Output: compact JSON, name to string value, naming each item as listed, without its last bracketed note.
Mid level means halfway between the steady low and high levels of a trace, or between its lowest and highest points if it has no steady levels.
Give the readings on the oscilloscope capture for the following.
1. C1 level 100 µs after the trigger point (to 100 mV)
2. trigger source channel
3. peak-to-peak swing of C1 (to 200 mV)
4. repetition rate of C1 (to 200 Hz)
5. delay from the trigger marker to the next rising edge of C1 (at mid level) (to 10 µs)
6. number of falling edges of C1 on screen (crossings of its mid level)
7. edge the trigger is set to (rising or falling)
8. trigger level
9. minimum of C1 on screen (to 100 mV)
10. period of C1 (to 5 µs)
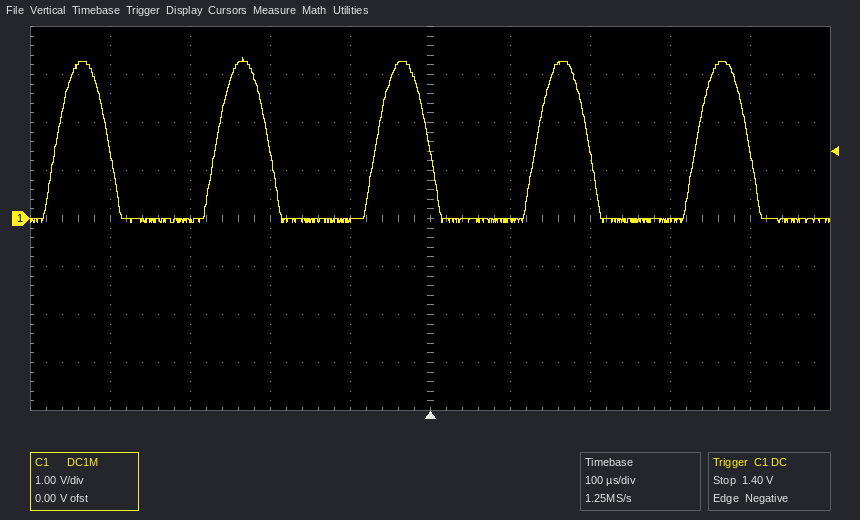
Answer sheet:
{"C1 level 100 µs after the trigger point": "0.0 V", "trigger source channel": "C1", "peak-to-peak swing of C1": "3.4 V", "repetition rate of C1": "5.0 kHz", "delay from the trigger marker to the next rising edge of C1 (at mid level)": "130 µs", "number of falling edges of C1 on screen": "5", "edge the trigger is set to": "falling", "trigger level": "1.40 V", "minimum of C1 on screen": "-100 mV", "period of C1": "200 µs"}
